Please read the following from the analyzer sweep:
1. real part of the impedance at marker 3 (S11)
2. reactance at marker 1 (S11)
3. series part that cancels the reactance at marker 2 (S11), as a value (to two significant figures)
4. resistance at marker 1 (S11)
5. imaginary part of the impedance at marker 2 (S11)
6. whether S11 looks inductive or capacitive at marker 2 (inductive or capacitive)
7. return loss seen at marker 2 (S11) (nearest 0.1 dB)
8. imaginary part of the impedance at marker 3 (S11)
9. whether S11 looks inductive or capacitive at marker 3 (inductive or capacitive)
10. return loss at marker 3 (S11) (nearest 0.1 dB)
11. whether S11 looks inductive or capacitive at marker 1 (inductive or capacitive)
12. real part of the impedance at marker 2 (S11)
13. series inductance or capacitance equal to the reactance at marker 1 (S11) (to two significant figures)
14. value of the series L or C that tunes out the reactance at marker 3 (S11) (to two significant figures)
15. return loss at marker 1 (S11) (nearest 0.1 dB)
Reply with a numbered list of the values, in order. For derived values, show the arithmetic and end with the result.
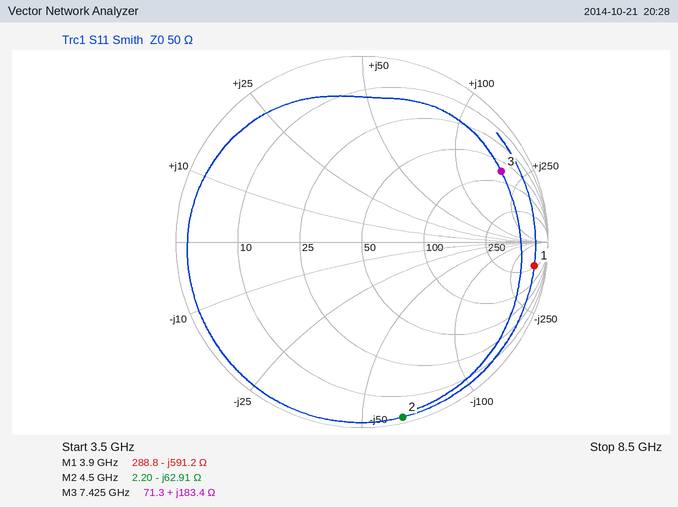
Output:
1. 71.3 Ω
2. -591.2 Ω
3. L = 62.91 Ω/(2π × 4.5 GHz) ≈ 2.2 nH
4. 288.8 Ω
5. -62.91 Ω
6. capacitive
7. 0.3 dB
8. +183.4 Ω
9. inductive
10. 1.5 dB
11. capacitive
12. 2.20 Ω
13. C = 1/(2π × 3.9 GHz × 591.2 Ω) ≈ 69 fF
14. C = 1/(2π × 7.425 GHz × 183.4 Ω) ≈ 117 fF, so 120 fF to two significant figures
15. 0.6 dB
